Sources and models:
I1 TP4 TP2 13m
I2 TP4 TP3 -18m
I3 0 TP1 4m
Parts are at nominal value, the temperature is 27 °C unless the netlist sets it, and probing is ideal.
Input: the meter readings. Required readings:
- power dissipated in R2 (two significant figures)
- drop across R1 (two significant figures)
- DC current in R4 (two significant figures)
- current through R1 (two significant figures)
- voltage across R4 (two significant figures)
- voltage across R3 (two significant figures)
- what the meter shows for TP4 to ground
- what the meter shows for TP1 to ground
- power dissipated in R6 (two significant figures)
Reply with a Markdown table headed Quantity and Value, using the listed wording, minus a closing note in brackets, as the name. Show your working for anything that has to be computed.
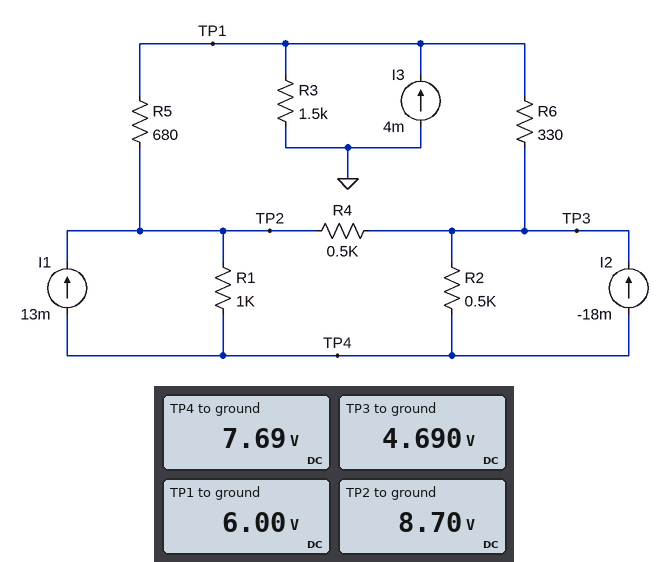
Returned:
| Quantity | Value |
|---|---|
| power dissipated in R2 | (7.69 V - 4.69 V)^2 / 500 Ω = 18 mW |
| drop across R1 | 8.7 V - 7.69 V = 1.0 V |
| DC current in R4 | (8.7 V - 4.69 V) / 500 Ω = 8.0 mA |
| current through R1 | (8.7 V - 7.69 V) / 1 kΩ = 1.0 mA |
| voltage across R4 | 8.7 V - 4.69 V = 4.0 V |
| voltage across R3 | 6 V = 6.0 V |
| what the meter shows for TP4 to ground | 7.69 V |
| what the meter shows for TP1 to ground | 6.00 V |
| power dissipated in R6 | (6 V - 4.69 V)^2 / 330 Ω = 5.2 mW |
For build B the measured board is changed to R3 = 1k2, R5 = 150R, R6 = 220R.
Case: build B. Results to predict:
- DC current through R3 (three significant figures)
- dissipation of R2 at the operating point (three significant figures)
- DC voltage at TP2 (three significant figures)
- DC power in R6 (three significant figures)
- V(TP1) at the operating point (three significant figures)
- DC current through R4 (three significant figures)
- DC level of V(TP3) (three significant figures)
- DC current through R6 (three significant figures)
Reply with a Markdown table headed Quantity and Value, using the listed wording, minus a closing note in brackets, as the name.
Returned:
| Quantity | Value |
|---|---|
| DC current through R3 | 4.00 mA |
| dissipation of R2 at the operating point | 13.3 mW |
| DC voltage at TP2 | 5.91 V |
| DC power in R6 | 12.0 mW |
| V(TP1) at the operating point | 4.80 V |
| DC current through R4 | 5.46 mA |
| DC level of V(TP3) | 3.18 V |
| DC current through R6 | 7.38 mA |
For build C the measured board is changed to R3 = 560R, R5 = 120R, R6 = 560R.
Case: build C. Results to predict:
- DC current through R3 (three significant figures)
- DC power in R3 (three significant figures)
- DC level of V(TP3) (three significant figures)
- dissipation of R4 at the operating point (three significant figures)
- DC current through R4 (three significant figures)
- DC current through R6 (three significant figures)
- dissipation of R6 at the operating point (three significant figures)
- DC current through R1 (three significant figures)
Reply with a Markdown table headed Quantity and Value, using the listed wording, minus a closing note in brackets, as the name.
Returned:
| Quantity | Value |
|---|---|
| DC current through R3 | 4.00 mA |
| DC power in R3 | 8.96 mW |
| DC level of V(TP3) | -679 mV |
| dissipation of R4 at the operating point | 25.1 mW |
| DC current through R4 | 7.09 mA |
| DC current through R6 | 5.21 mA |
| dissipation of R6 at the operating point | 15.2 mW |
| DC current through R1 | 697 µA |
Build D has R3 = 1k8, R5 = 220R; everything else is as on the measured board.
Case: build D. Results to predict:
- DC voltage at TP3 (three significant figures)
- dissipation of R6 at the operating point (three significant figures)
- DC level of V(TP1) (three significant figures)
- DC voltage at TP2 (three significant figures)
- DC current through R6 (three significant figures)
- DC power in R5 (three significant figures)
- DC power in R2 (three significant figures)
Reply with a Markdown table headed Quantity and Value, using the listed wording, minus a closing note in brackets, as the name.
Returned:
| Quantity | Value |
|---|---|
| DC voltage at TP3 | 5.24 V |
| dissipation of R6 at the operating point | 11.7 mW |
| DC level of V(TP1) | 7.20 V |
| DC voltage at TP2 | 8.51 V |
| DC current through R6 | 5.95 mA |
| DC power in R5 | 7.78 mW |
| DC power in R2 | 15.2 mW |
